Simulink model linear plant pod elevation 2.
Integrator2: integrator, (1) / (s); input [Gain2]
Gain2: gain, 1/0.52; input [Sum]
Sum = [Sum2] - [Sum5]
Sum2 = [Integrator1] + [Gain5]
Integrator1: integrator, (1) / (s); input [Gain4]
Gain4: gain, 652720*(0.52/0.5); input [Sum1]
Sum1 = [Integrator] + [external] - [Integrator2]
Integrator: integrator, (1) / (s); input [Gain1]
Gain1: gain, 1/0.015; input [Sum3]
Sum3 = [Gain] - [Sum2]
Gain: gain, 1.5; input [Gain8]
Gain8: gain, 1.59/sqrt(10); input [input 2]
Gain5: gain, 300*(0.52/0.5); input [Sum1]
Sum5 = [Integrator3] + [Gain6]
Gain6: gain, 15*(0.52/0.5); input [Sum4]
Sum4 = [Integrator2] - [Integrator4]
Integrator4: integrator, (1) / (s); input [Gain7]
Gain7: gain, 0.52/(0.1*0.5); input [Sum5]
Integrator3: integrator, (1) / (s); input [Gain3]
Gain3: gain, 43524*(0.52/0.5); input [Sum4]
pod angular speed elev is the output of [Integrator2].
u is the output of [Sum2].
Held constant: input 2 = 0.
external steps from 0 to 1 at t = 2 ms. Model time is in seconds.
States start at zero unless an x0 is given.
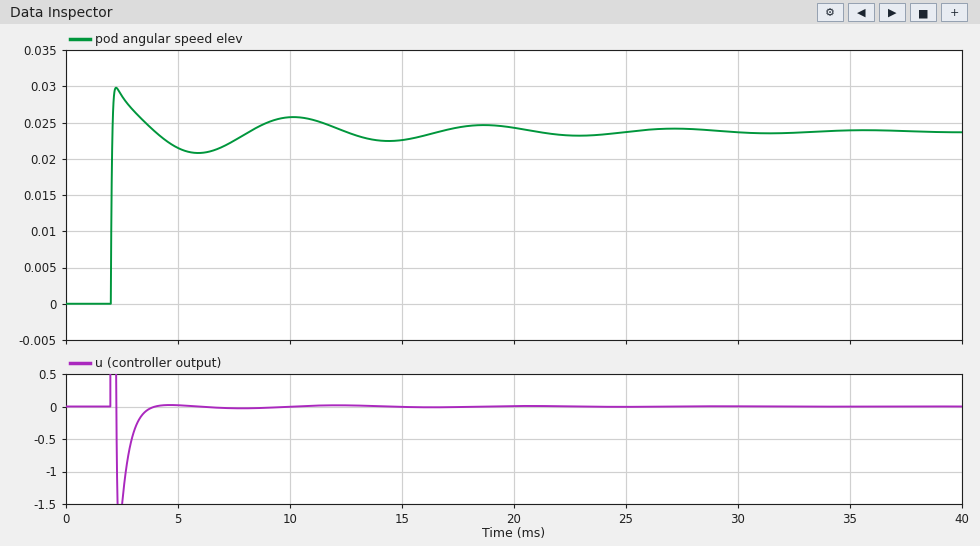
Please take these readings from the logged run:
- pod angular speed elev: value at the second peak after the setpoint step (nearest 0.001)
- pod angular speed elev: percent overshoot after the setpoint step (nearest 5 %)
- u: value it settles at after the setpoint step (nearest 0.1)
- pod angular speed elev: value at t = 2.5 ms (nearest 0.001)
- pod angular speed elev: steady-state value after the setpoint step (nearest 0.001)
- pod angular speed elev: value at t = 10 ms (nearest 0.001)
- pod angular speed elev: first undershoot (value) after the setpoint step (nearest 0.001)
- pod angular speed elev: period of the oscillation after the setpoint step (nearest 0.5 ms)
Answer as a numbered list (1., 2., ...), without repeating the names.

1. 0.026
2. 25 %
3. 0.0
4. 0.029
5. 0.024
6. 0.026
7. 0.021
8. 8.0 ms
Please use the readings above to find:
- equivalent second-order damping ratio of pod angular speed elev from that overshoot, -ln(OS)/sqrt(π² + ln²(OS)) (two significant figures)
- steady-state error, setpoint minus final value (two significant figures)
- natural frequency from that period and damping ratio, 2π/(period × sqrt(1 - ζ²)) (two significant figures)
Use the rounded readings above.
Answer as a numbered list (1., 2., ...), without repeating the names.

1. 0.40
2. 0.98
3. 0.86 rad/ms
